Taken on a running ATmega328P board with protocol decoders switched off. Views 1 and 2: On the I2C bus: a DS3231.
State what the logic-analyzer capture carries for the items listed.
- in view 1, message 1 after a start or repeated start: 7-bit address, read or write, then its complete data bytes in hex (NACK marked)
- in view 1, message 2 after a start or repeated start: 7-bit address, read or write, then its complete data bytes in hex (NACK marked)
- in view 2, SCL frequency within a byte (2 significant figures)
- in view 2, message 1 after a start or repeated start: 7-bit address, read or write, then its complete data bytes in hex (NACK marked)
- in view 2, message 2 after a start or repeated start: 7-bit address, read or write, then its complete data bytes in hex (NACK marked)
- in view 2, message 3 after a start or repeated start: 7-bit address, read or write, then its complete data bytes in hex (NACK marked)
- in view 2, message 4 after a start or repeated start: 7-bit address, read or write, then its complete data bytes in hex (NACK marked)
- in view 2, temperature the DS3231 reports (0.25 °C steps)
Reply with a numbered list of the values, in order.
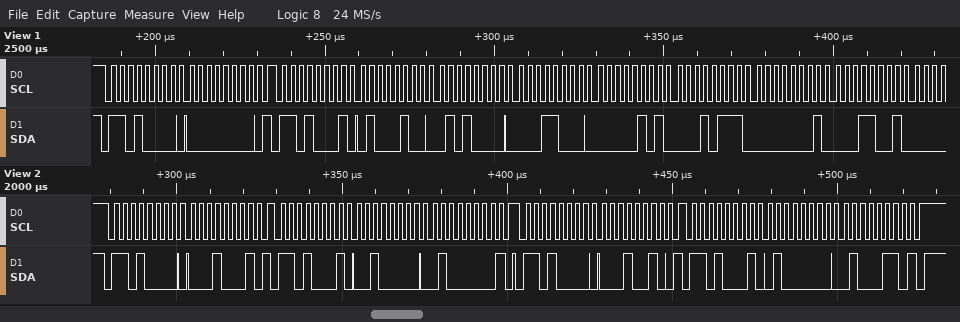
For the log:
1. 0x68 write: 00
2. 0x68 read: 44 50 18 05 17 01 19
3. 400 kHz
4. 0x68 write: 11
5. 0x68 read: 20 40 NACK
6. 0x68 write: 12
7. 0x68 read: 40 46 NACK
8. 32.25 °C
